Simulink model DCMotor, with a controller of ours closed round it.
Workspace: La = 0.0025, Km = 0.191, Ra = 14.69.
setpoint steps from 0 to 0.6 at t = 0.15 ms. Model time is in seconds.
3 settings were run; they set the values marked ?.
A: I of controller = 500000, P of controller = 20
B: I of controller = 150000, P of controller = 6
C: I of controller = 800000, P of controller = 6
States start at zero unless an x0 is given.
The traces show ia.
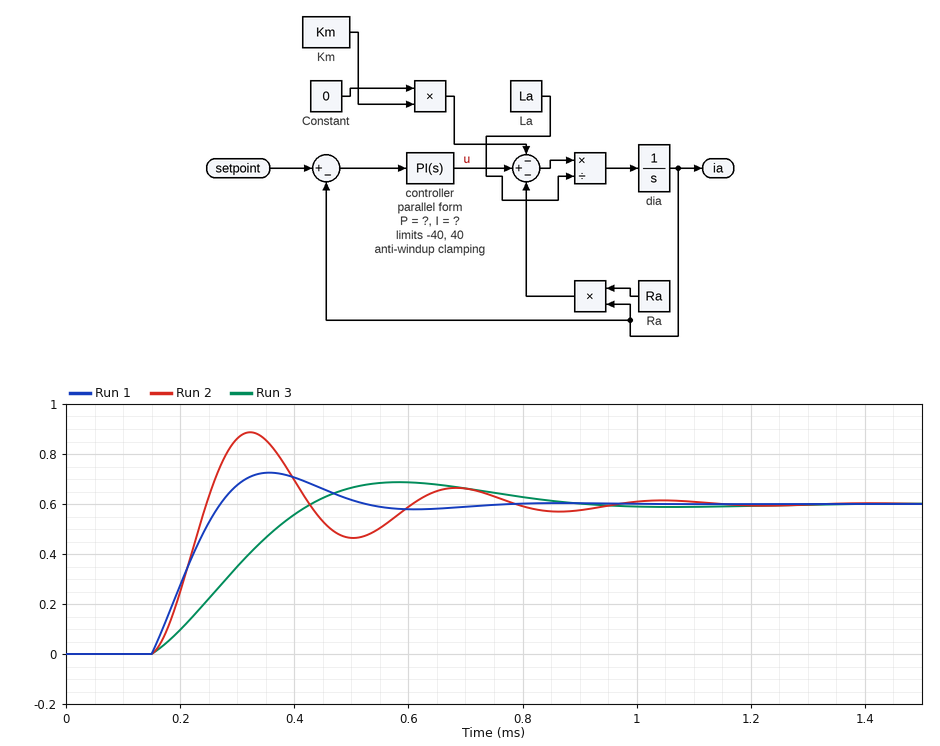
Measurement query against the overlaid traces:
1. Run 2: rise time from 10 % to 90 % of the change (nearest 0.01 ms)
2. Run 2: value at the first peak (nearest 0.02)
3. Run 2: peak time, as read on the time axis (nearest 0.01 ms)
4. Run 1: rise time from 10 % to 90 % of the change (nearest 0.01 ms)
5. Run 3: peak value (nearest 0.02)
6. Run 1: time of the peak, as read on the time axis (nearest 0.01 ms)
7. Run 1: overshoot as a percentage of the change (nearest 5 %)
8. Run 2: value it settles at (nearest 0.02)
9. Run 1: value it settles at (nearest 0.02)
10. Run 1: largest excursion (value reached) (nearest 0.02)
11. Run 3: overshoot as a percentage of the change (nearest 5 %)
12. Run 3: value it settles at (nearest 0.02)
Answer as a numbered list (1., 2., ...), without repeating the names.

1. 0.07 ms
2. 0.88
3. 0.32 ms
4. 0.09 ms
5. 0.68
6. 0.36 ms
7. 20 %
8. 0.60
9. 0.60
10. 0.72
11. 15 %
12. 0.60
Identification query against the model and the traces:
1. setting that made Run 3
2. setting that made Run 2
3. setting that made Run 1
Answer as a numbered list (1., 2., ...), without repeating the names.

1. B
2. C
3. A
